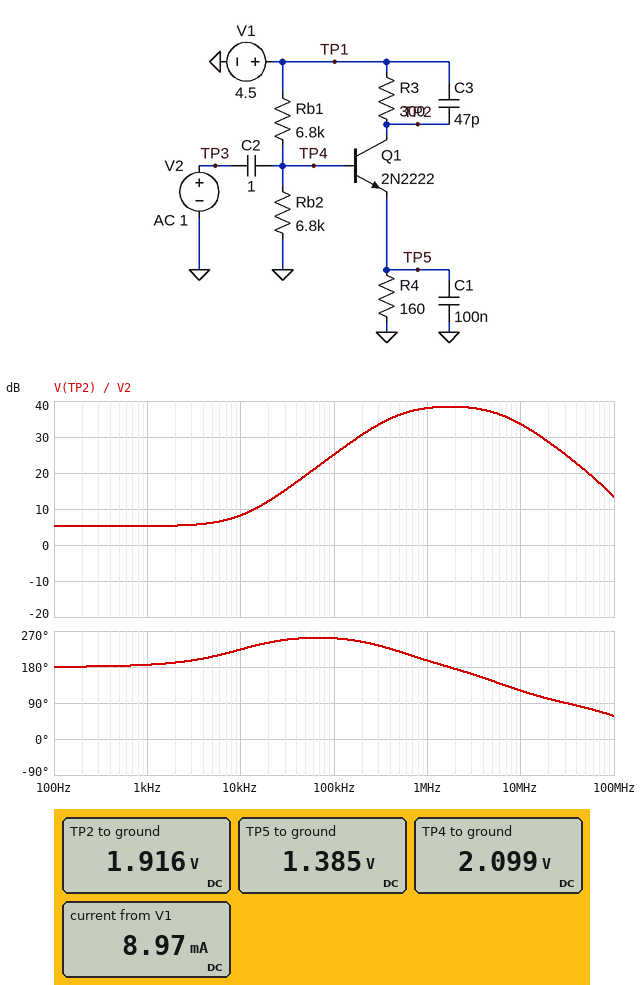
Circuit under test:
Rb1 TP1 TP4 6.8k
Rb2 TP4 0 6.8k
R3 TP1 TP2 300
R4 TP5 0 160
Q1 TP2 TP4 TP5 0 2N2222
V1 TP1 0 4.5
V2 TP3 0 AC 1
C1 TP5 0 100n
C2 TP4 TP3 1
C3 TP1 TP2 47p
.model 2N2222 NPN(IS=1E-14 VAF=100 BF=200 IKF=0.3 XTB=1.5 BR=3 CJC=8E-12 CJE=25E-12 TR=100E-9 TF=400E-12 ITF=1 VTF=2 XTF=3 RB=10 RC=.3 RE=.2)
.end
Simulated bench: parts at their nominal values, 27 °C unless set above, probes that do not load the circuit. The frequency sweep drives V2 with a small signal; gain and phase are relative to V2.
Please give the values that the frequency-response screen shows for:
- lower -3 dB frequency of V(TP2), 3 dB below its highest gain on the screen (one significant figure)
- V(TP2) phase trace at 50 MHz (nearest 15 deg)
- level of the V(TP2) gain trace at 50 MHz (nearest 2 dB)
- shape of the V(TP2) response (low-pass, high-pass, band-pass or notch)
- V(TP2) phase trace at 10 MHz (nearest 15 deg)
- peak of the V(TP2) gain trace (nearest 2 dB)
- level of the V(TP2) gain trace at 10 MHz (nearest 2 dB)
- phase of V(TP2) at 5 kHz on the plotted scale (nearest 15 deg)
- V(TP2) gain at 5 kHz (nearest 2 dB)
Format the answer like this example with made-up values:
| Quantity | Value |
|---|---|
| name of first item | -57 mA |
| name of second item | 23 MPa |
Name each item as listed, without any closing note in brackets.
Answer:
| Quantity | Value |
|---|---|
| lower -3 dB frequency of V(TP2), 3 dB below its highest gain on the screen | 400 kHz |
| V(TP2) phase trace at 50 MHz | 75 deg |
| level of the V(TP2) gain trace at 50 MHz | 20 dB |
| shape of the V(TP2) response | band-pass |
| V(TP2) phase trace at 10 MHz | 120 deg |
| peak of the V(TP2) gain trace | 38 dB |
| level of the V(TP2) gain trace at 10 MHz | 34 dB |
| phase of V(TP2) at 5 kHz on the plotted scale | 210 deg |
| V(TP2) gain at 5 kHz | 6 dB |
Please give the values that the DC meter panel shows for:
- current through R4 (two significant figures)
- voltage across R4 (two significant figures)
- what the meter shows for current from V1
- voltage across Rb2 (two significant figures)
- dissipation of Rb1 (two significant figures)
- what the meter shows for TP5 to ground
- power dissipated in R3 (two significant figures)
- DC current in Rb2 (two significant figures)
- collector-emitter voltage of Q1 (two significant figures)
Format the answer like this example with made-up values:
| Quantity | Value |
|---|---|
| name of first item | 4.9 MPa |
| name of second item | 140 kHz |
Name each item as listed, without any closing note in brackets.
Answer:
| Quantity | Value |
|---|---|
| current through R4 | 8.7 mA |
| voltage across R4 | 1.4 V |
| what the meter shows for current from V1 | 8.97 mA |
| voltage across Rb2 | 2.1 V |
| dissipation of Rb1 | 850 µW |
| what the meter shows for TP5 to ground | 1.385 V |
| power dissipated in R3 | 22 mW |
| DC current in Rb2 | 310 µA |
| collector-emitter voltage of Q1 | 530 mV |
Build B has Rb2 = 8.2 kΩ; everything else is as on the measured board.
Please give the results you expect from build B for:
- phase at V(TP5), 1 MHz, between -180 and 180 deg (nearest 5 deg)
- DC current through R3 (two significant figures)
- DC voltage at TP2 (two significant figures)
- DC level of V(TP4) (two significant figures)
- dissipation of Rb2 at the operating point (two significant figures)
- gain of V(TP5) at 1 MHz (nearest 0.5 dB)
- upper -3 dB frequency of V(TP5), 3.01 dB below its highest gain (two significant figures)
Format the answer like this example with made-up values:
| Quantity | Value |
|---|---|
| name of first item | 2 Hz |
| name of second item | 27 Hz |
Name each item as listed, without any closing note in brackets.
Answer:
| Quantity | Value |
|---|---|
| phase at V(TP5), 1 MHz, between -180 and 180 deg | -90 deg |
| DC current through R3 | 9.4 mA |
| DC voltage at TP2 | 1.7 V |
| DC level of V(TP4) | 2.2 V |
| dissipation of Rb2 at the operating point | 610 µW |
| gain of V(TP5) at 1 MHz | -11.0 dB |
| upper -3 dB frequency of V(TP5), 3.01 dB below its highest gain | 340 kHz |
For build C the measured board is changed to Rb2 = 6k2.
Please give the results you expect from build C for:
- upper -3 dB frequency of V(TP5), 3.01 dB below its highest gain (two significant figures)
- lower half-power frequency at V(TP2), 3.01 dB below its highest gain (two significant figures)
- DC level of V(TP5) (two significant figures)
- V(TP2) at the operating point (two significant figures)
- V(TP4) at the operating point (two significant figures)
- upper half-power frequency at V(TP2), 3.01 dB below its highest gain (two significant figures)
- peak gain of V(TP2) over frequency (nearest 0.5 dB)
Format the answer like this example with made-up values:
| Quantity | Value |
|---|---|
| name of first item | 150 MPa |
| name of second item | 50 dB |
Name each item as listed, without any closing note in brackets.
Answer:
| Quantity | Value |
|---|---|
| upper -3 dB frequency of V(TP5), 3.01 dB below its highest gain | 460 kHz |
| lower half-power frequency at V(TP2), 3.01 dB below its highest gain | 410 kHz |
| DC level of V(TP5) | 1.3 V |
| V(TP2) at the operating point | 2.1 V |
| V(TP4) at the operating point | 2.0 V |
| upper half-power frequency at V(TP2), 3.01 dB below its highest gain | 7.6 MHz |
| peak gain of V(TP2) over frequency | 38.0 dB |
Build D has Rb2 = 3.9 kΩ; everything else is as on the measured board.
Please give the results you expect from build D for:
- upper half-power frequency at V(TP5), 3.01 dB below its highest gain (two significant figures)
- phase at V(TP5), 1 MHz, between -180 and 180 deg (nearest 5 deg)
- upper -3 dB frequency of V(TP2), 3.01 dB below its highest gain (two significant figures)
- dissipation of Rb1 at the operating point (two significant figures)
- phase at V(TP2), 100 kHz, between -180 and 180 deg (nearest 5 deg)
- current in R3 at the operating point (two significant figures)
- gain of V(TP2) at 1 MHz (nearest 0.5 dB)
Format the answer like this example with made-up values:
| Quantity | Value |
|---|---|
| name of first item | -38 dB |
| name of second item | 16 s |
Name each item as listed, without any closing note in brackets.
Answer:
| Quantity | Value |
|---|---|
| upper half-power frequency at V(TP5), 3.01 dB below its highest gain | 320 kHz |
| phase at V(TP5), 1 MHz, between -180 and 180 deg | -75 deg |
| upper -3 dB frequency of V(TP2), 3.01 dB below its highest gain | 8.9 MHz |
| dissipation of Rb1 at the operating point | 1.3 mW |
| phase at V(TP2), 100 kHz, between -180 and 180 deg | -115 deg |
| current in R3 at the operating point | 5.4 mA |
| gain of V(TP2) at 1 MHz | 35.0 dB |
